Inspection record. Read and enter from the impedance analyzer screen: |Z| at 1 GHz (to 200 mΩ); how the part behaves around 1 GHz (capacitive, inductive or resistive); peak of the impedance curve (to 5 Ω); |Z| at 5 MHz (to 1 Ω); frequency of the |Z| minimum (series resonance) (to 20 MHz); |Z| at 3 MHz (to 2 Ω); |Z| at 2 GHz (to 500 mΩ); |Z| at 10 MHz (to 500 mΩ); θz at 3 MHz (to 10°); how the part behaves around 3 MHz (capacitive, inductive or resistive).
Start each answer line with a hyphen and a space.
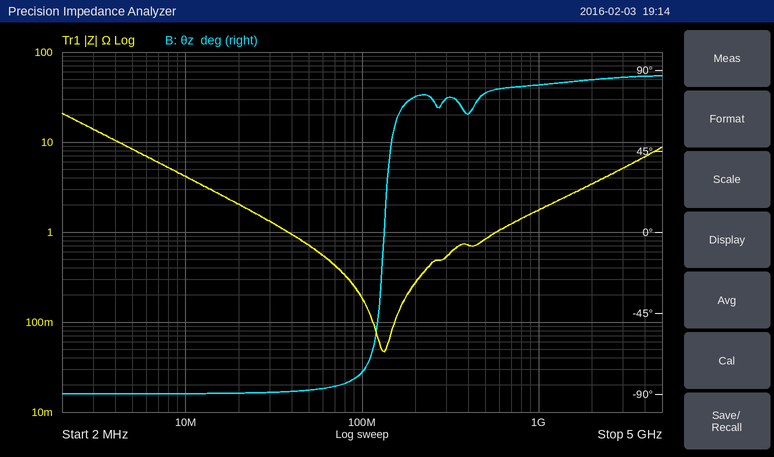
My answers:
- 1.8 Ω
- inductive
- 20 Ω
- 8 Ω
- 140 MHz
- 14 Ω
- 3.5 Ω
- 4.0 Ω
- -90°
- capacitive
